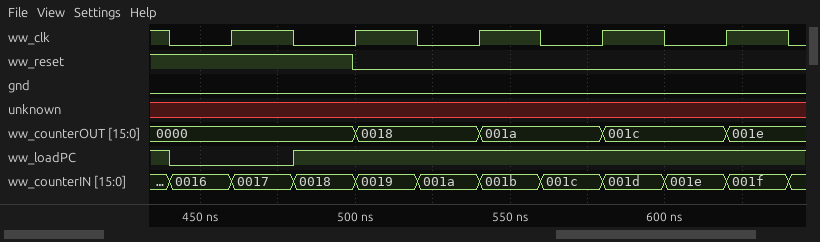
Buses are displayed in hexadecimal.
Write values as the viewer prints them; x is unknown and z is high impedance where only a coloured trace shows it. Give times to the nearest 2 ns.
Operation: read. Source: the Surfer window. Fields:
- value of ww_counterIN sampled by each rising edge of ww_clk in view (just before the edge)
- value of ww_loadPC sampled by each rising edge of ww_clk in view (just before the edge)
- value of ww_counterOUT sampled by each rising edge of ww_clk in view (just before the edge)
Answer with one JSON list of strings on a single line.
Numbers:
["0016, 0018, 001a, 001c, 001e", "0 1 1 1 1", "0000, 0000, 0018, 001a, 001c"]
